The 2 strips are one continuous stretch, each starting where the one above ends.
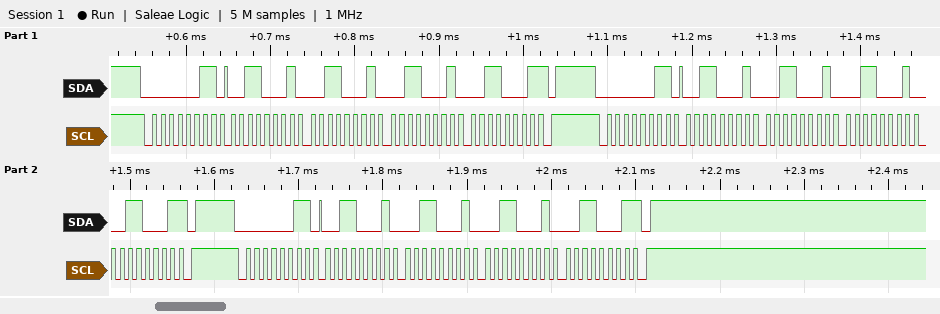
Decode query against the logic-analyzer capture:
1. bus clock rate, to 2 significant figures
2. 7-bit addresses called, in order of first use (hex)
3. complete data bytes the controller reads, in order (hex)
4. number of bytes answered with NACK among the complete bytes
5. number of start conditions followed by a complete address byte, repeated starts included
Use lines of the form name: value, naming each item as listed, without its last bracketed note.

bus clock rate, to 2 significant figures: 100 kHz
7-bit addresses called, in order of first use: 0x01
complete data bytes the controller reads, in order: 31 31 31 31 31 31 31 31 31 31 31 31
number of bytes answered with NACK among the complete bytes: 3
number of start conditions followed by a complete address byte, repeated starts included: 3
